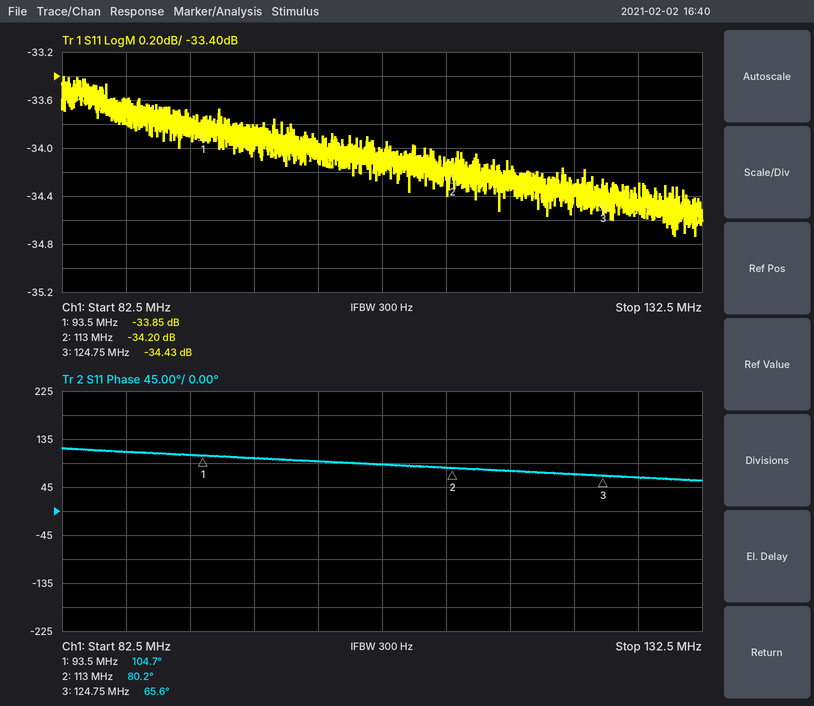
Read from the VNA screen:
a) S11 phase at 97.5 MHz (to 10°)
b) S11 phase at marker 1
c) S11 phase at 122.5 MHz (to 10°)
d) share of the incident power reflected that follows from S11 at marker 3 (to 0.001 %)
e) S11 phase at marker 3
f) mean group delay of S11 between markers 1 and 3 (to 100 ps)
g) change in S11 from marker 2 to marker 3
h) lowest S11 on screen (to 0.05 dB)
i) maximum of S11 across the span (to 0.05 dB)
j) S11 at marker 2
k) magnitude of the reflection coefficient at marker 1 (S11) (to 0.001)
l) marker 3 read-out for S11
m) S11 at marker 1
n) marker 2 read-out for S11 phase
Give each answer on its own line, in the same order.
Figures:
100°
104.7°
70°
0.036 %
65.6°
3.5 ns
-0.23 dB
-34.75 dB
-33.40 dB
-34.20 dB
0.020
-34.43 dB
-33.85 dB
80.2°
